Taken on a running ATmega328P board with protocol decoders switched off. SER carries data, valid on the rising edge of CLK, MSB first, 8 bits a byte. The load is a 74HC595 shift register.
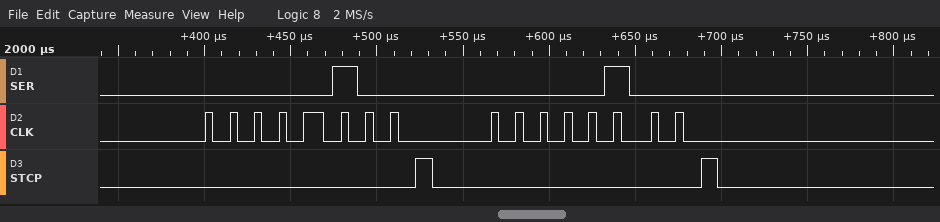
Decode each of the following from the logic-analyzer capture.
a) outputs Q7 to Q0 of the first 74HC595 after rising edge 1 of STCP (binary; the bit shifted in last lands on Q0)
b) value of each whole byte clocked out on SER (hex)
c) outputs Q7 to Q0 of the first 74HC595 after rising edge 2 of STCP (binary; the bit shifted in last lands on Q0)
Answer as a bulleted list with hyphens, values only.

- 00000100
- 04 04
- 00000100
